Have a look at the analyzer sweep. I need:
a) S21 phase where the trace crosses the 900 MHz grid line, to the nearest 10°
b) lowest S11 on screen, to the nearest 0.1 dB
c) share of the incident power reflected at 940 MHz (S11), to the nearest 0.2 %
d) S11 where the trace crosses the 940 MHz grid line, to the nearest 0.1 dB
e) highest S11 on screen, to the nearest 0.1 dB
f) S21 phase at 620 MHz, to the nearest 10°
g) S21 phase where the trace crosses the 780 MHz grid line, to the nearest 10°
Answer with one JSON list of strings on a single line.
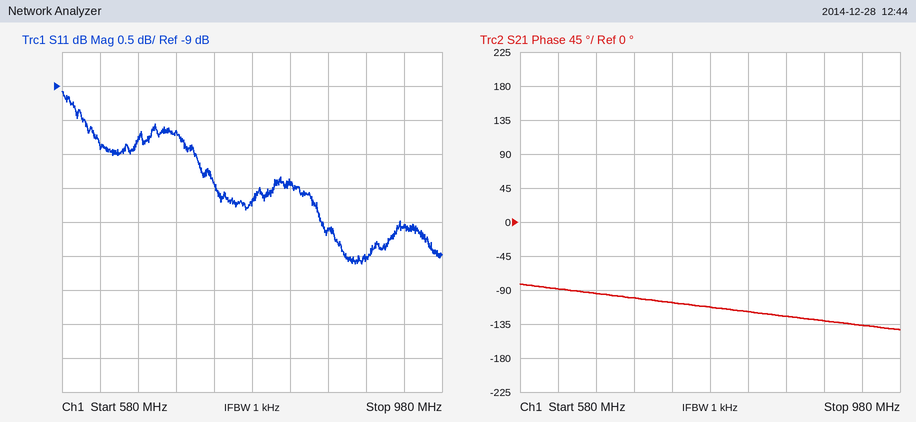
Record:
["-130°", "-11.6 dB", "7.8 %", "-11.1 dB", "-9.1 dB", "-90°", "-110°"]
